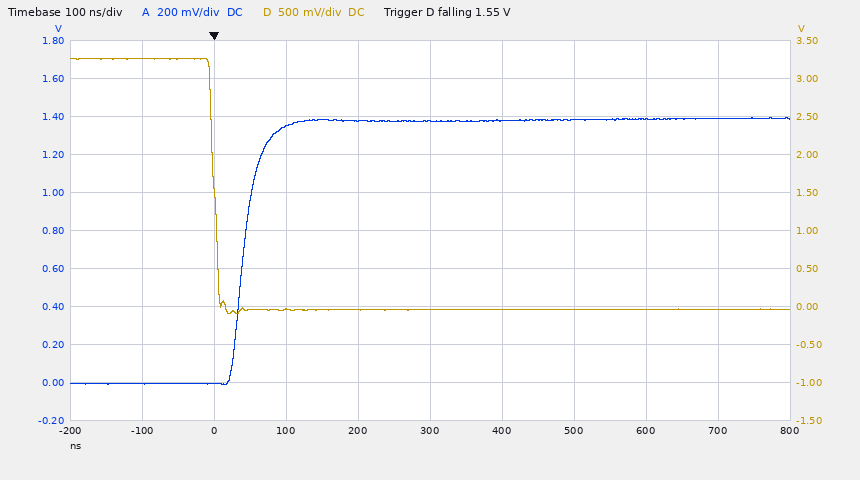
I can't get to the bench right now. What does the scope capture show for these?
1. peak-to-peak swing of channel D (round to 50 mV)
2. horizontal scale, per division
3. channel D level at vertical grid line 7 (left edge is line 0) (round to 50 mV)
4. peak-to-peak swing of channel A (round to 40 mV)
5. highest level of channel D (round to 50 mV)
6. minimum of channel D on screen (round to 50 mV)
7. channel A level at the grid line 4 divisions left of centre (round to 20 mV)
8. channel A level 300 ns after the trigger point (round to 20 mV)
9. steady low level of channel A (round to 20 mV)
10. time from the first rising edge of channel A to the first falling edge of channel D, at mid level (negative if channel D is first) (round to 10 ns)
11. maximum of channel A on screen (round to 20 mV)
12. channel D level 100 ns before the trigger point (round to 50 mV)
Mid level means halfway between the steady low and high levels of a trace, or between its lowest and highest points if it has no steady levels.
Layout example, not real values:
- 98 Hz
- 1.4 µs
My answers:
- 3.35 V
- 100 ns
- -50 mV
- 1.40 V
- 3.25 V
- -100 mV
- 0 mV
- 1.38 V
- 0 mV
- -40 ns
- 1.40 V
- 3.25 V
